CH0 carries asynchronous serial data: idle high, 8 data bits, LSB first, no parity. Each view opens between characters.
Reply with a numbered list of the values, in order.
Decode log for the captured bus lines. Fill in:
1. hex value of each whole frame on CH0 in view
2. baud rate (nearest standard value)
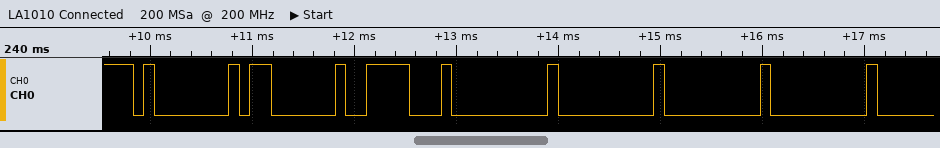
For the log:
1. 01, 03, 1E, 00, 00, 00, 00
2. 9600 baud
